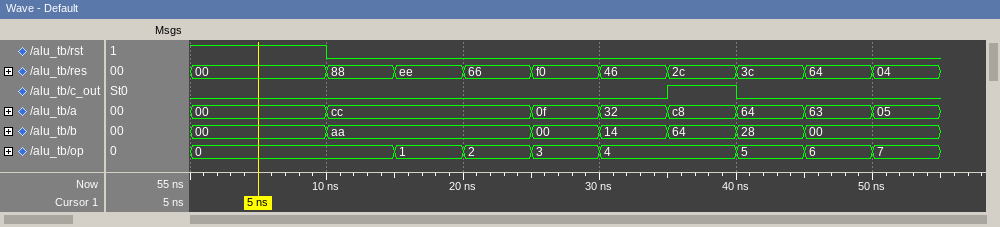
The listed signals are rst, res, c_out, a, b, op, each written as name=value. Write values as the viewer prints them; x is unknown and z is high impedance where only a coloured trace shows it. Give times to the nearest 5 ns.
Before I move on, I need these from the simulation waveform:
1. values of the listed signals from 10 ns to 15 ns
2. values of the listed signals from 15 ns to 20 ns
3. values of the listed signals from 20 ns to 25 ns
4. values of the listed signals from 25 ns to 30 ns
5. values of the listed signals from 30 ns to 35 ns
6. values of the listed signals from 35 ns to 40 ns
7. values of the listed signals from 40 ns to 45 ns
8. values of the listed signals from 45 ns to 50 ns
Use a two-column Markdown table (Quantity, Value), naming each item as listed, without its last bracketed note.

| Quantity | Value |
|---|---|
| values of the listed signals from 10 ns to 15 ns | rst=0, res=88, c_out=0, a=cc, b=aa, op=0 |
| values of the listed signals from 15 ns to 20 ns | rst=0, res=ee, c_out=0, a=cc, b=aa, op=1 |
| values of the listed signals from 20 ns to 25 ns | rst=0, res=66, c_out=0, a=cc, b=aa, op=2 |
| values of the listed signals from 25 ns to 30 ns | rst=0, res=f0, c_out=0, a=0f, b=00, op=3 |
| values of the listed signals from 30 ns to 35 ns | rst=0, res=46, c_out=0, a=32, b=14, op=4 |
| values of the listed signals from 35 ns to 40 ns | rst=0, res=2c, c_out=1, a=c8, b=64, op=4 |
| values of the listed signals from 40 ns to 45 ns | rst=0, res=3c, c_out=0, a=64, b=28, op=5 |
| values of the listed signals from 45 ns to 50 ns | rst=0, res=64, c_out=0, a=63, b=00, op=6 |
